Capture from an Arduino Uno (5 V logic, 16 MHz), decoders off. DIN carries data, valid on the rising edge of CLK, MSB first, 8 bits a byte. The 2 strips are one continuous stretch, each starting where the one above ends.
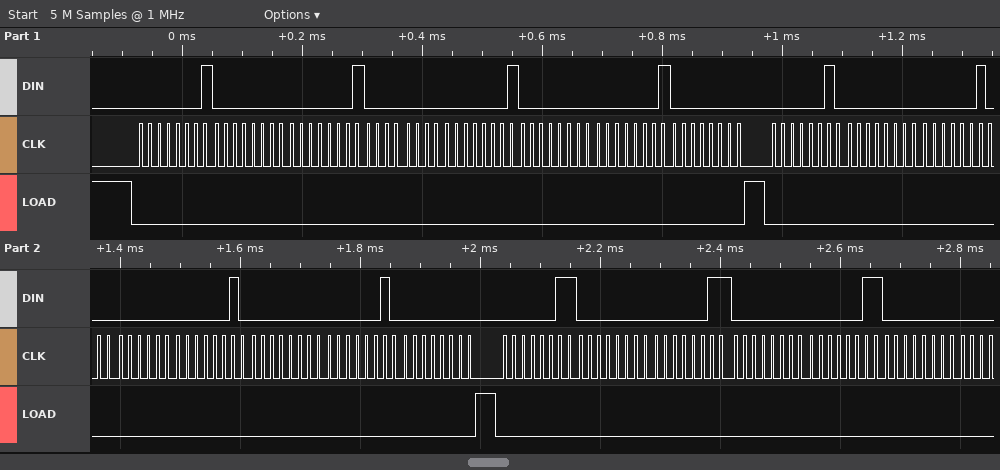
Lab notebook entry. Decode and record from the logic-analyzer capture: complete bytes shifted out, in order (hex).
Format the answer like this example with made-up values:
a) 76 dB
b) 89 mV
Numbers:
a) 0x01 0x00 0x01 0x00 0x01 0x00 0x01 0x00 0x02 0x00 0x02 0x00 0x02 0x00 0x02 0x00 0x03 0x00 0x03 0x00 0x03 0x00
